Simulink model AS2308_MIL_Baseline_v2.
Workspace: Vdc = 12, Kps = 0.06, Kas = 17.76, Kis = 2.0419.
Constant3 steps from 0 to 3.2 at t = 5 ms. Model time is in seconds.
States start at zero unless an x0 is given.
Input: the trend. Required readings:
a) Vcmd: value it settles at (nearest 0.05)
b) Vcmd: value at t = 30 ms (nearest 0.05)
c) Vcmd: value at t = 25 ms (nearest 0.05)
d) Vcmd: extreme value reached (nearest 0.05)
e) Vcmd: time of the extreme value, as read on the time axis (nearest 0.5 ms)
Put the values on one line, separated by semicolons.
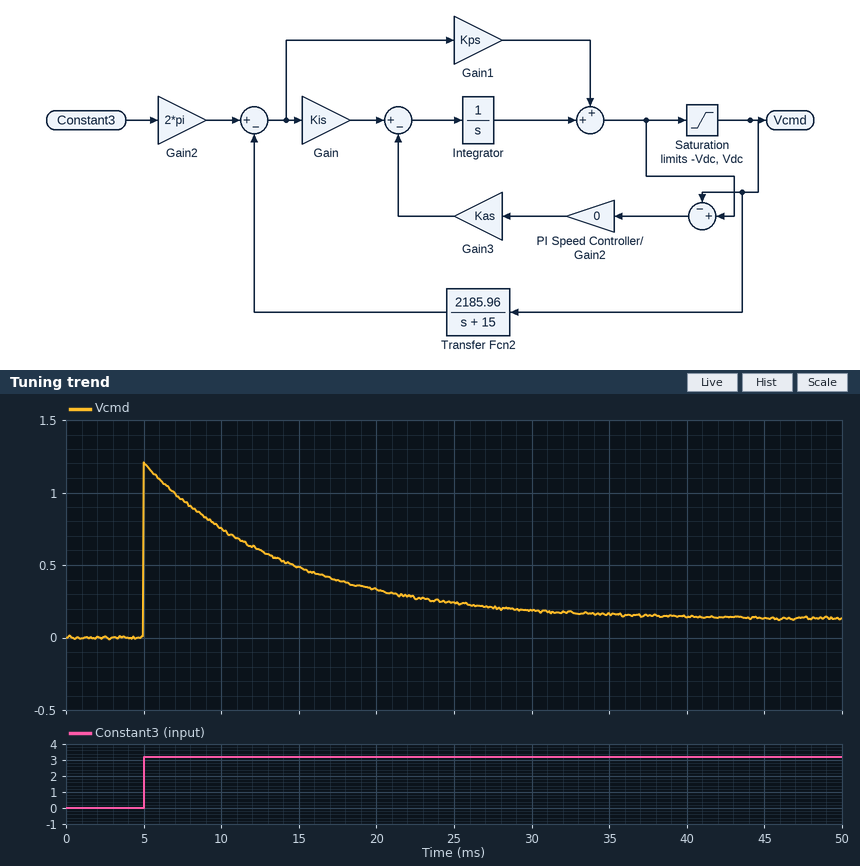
0.15; 0.20; 0.25; 1.20; 5.0 ms
